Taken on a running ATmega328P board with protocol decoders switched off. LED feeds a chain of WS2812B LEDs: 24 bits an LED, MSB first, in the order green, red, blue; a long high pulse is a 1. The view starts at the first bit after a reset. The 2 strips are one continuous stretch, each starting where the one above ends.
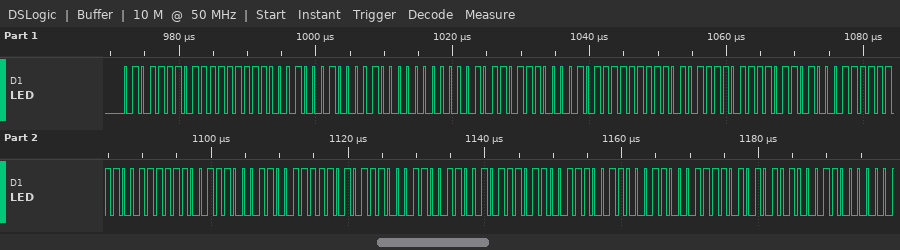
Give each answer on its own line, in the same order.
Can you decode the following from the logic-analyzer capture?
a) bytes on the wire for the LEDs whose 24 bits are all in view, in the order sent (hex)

5E FF 88 84 00 5B 85 FF 5E F6 8F F3 F3 8C FA E3 32 EC E6 31 EA
